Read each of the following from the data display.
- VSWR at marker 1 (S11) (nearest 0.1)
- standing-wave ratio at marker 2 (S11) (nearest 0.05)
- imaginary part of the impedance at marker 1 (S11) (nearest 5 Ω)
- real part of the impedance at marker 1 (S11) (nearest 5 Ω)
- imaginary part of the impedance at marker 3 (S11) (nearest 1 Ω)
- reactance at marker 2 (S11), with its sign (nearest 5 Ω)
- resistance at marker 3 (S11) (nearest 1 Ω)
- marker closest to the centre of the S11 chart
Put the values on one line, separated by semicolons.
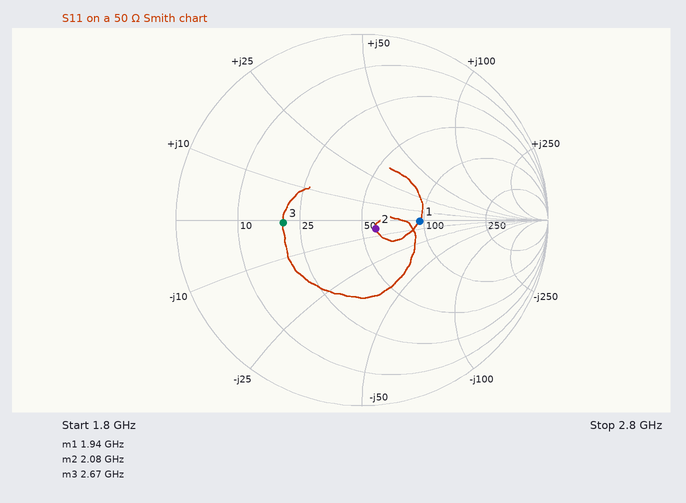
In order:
1.9; 1.20; 0 Ω; 95 Ω; -1 Ω; -5 Ω; 20 Ω; marker 2
